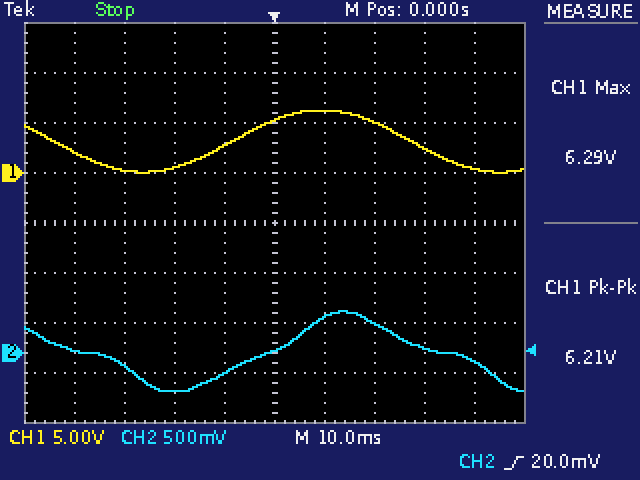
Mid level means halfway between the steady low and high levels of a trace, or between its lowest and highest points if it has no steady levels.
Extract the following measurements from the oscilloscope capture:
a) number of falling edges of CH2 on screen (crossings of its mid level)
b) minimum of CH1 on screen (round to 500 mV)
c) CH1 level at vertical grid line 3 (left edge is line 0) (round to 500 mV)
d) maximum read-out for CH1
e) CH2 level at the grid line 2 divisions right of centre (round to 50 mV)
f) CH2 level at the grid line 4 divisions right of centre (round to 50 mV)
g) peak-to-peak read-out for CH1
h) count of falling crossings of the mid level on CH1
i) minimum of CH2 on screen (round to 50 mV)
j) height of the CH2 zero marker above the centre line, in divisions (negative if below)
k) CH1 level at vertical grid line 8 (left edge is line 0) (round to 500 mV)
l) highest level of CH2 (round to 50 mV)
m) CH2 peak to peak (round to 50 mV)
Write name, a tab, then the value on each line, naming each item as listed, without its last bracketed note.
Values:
number of falling edges of CH2 on screen	2
minimum of CH1 on screen	0.0 V
CH1 level at vertical grid line 3 (left edge is line 0)	500 mV
maximum read-out for CH1	6.29 V
CH2 level at the grid line 2 divisions right of centre	300 mV
CH2 level at the grid line 4 divisions right of centre	-100 mV
peak-to-peak read-out for CH1	6.21 V
count of falling crossings of the mid level on CH1	2
minimum of CH2 on screen	-400 mV
height of the CH2 zero marker above the centre line, in divisions	-2.6 div
CH1 level at vertical grid line 8 (left edge is line 0)	2.5 V
highest level of CH2	400 mV
CH2 peak to peak	800 mV
